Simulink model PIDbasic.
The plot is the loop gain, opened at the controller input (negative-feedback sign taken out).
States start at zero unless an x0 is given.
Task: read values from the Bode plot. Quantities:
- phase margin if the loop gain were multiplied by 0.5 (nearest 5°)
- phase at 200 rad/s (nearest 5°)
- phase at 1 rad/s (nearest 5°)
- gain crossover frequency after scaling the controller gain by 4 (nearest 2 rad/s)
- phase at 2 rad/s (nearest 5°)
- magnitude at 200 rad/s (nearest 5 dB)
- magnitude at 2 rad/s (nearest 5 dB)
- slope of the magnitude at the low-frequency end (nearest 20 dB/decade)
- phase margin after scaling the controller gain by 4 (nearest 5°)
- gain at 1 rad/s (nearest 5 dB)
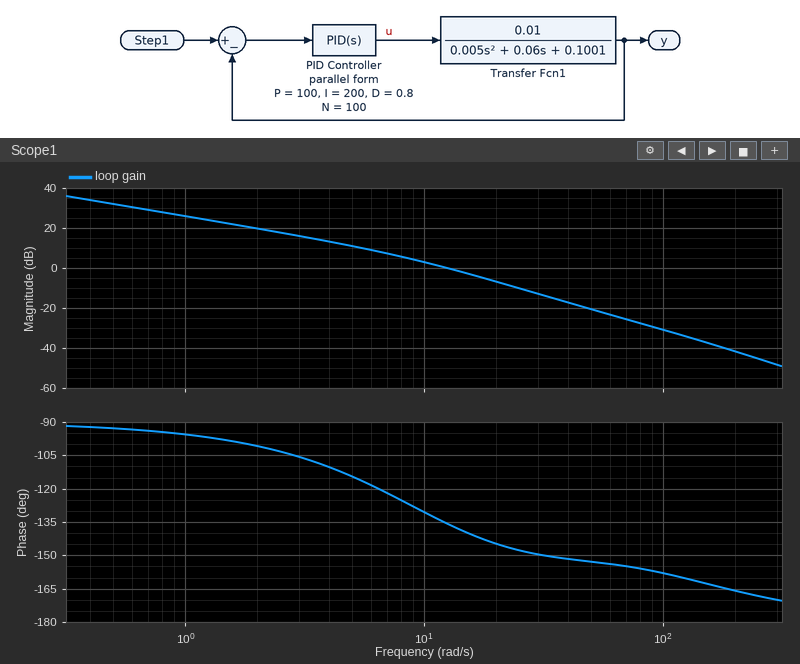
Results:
55°
-165°
-95°
28 rad/s
-100°
-40 dB
20 dB
-20 dB/decade
30°
25 dB
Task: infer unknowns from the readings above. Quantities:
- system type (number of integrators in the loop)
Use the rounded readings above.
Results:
1
